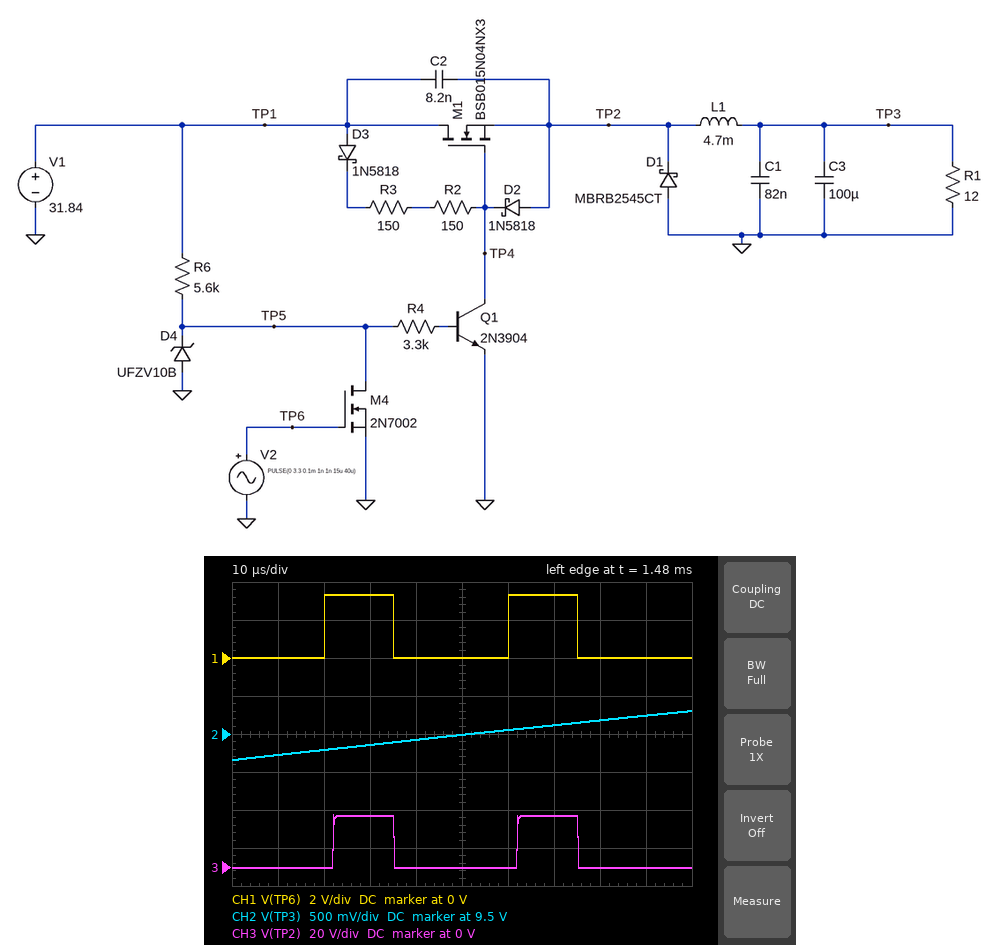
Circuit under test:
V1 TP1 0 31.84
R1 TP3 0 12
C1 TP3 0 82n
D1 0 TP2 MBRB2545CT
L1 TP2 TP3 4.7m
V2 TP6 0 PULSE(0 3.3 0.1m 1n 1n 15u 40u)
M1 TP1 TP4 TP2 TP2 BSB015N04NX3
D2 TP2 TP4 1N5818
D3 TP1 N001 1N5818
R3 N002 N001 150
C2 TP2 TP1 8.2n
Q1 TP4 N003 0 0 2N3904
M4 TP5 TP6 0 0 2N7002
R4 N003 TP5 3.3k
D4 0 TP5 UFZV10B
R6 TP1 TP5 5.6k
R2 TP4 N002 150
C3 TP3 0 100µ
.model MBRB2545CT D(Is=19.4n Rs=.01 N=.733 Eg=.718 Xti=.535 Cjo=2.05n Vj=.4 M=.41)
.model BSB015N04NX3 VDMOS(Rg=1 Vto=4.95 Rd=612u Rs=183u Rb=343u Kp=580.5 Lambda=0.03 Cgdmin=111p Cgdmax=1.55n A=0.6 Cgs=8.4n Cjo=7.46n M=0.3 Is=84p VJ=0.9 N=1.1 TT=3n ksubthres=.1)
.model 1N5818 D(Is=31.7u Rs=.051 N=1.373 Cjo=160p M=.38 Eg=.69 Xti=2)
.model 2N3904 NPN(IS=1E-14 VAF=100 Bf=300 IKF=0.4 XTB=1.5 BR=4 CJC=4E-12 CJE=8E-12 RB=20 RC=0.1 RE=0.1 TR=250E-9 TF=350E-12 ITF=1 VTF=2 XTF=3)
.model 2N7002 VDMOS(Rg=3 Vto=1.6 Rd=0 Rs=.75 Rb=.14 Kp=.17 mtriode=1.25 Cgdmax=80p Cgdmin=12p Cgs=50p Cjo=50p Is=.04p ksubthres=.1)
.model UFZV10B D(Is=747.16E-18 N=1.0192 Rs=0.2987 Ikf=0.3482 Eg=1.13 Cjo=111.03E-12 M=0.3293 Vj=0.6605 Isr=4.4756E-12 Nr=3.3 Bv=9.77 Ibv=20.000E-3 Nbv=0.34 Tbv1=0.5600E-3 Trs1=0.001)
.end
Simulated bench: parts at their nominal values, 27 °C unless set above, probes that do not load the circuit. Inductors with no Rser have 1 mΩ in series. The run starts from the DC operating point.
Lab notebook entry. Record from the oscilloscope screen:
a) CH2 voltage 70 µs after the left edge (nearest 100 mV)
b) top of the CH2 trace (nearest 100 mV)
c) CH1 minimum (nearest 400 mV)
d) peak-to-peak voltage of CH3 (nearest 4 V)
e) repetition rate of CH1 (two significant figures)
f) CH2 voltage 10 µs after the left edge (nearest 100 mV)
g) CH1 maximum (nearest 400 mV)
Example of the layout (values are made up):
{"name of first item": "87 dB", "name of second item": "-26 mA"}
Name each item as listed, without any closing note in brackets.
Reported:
{"CH2 voltage 70 µs after the left edge": "9.6 V", "top of the CH2 trace": "9.8 V", "CH1 minimum": "0 V", "peak-to-peak voltage of CH3": "28 V", "repetition rate of CH1": "25 kHz", "CH2 voltage 10 µs after the left edge": "9.2 V", "CH1 maximum": "3.2 V"}
